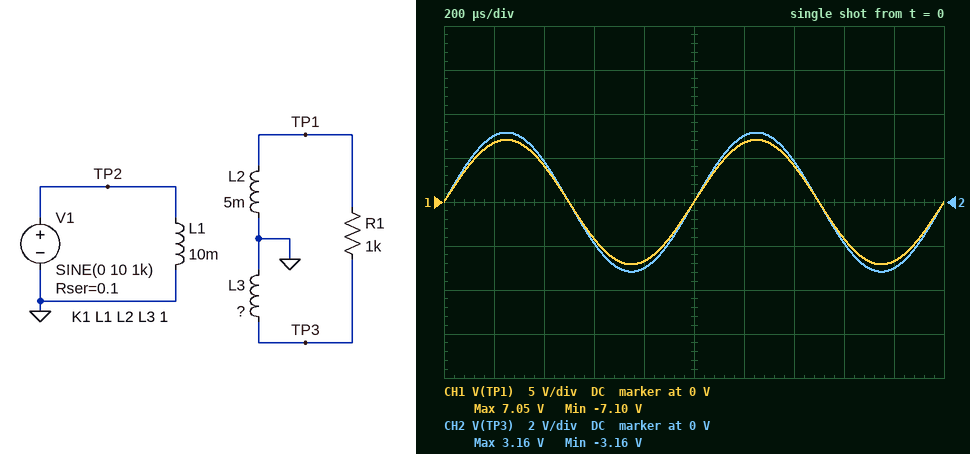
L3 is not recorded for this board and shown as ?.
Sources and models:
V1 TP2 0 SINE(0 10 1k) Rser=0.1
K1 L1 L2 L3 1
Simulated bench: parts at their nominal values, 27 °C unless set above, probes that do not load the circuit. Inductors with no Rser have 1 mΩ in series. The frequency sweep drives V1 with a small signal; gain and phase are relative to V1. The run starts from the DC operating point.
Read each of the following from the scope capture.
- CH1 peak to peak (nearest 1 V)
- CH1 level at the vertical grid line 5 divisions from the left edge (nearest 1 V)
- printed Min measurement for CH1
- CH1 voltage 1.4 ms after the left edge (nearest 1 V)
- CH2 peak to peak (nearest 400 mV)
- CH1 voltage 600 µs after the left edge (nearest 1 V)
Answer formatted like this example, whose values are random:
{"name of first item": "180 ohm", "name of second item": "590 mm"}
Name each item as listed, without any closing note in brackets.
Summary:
{"CH1 peak to peak": "14 V", "CH1 level at the vertical grid line 5 divisions from the left edge": "0 V", "printed Min measurement for CH1": "-7.10 V", "CH1 voltage 1.4 ms after the left edge": "4 V", "CH2 peak to peak": "6.4 V", "CH1 voltage 600 µs after the left edge": "-4 V"}
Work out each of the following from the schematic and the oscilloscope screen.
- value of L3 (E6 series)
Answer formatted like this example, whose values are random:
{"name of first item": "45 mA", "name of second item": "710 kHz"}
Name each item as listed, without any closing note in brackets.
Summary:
{"value of L3": "1 mH"}
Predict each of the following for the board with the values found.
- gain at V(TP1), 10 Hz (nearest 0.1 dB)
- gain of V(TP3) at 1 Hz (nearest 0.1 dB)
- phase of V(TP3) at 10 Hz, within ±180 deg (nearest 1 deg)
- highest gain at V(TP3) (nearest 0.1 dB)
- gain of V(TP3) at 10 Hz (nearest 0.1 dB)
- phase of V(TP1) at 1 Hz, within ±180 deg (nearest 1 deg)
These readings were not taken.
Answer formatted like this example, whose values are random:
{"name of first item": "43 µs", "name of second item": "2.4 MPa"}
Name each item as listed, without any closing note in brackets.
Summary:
{"gain at V(TP1), 10 Hz": "-3.1 dB", "gain of V(TP3) at 1 Hz": "-15.5 dB", "phase of V(TP3) at 10 Hz, within ±180 deg": "9 deg", "highest gain at V(TP3)": "-10.0 dB", "gain of V(TP3) at 10 Hz": "-10.1 dB", "phase of V(TP1) at 1 Hz, within ±180 deg": "58 deg"}
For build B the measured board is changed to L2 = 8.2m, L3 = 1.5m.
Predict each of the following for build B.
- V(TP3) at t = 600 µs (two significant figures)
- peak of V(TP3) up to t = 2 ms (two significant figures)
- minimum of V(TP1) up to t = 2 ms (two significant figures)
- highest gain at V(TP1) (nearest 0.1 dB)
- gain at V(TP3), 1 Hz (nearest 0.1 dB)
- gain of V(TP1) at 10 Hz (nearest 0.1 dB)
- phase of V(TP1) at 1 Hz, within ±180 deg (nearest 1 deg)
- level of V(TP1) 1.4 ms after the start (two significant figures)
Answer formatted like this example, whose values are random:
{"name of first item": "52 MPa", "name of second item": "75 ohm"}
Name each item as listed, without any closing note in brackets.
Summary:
{"V(TP3) at t = 600 µs": "-2.3 V", "peak of V(TP3) up to t = 2 ms": "3.9 V", "minimum of V(TP1) up to t = 2 ms": "-9.1 V", "highest gain at V(TP1)": "-0.9 dB", "gain at V(TP3), 1 Hz": "-13.8 dB", "gain of V(TP1) at 10 Hz": "-1.0 dB", "phase of V(TP1) at 1 Hz, within ±180 deg": "58 deg", "level of V(TP1) 1.4 ms after the start": "5.3 V"}
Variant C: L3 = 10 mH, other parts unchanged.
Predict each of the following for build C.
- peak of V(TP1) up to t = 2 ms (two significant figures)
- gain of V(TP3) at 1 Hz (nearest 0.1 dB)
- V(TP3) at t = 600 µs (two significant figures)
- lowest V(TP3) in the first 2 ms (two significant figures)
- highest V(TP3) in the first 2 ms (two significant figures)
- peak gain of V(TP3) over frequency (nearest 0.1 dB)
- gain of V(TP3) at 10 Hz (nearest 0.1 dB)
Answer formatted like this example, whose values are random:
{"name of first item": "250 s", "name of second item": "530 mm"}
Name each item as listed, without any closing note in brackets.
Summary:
{"peak of V(TP1) up to t = 2 ms": "7.1 V", "gain of V(TP3) at 1 Hz": "-5.5 dB", "V(TP3) at t = 600 µs": "-5.9 V", "lowest V(TP3) in the first 2 ms": "-10 V", "highest V(TP3) in the first 2 ms": "10 V", "peak gain of V(TP3) over frequency": "0 dB", "gain of V(TP3) at 10 Hz": "-0.1 dB"}
